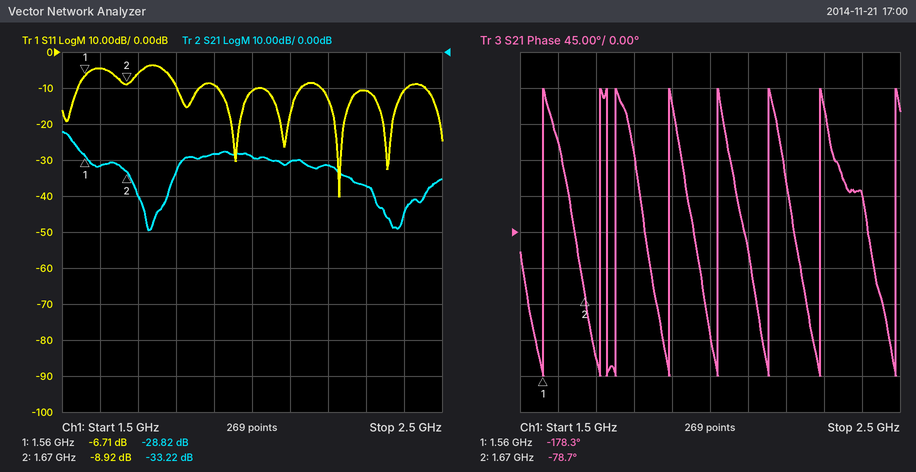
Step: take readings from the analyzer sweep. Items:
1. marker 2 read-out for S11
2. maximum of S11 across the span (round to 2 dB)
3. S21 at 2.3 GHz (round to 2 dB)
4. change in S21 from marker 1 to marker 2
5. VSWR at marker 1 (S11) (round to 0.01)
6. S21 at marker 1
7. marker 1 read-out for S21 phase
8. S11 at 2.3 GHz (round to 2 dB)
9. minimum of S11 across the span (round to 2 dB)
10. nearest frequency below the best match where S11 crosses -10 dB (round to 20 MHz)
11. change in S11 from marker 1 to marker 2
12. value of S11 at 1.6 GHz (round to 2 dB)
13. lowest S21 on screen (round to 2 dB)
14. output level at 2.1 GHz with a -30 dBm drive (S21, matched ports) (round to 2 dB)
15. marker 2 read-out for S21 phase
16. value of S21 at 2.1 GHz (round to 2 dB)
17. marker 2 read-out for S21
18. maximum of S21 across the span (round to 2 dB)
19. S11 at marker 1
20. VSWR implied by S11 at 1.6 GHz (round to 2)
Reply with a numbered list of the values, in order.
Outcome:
1. -8.92 dB
2. -4 dB
3. -38 dB
4. -4.40 dB
5. 2.72
6. -28.82 dB
7. -178.3°
8. -10 dB
9. -40 dB
10. 2.18 GHz
11. -2.21 dB
12. -4 dB
13. -50 dB
14. -60 dBm
15. -78.7°
16. -30 dB
17. -33.22 dB
18. -22 dB
19. -6.71 dB
20. 4
